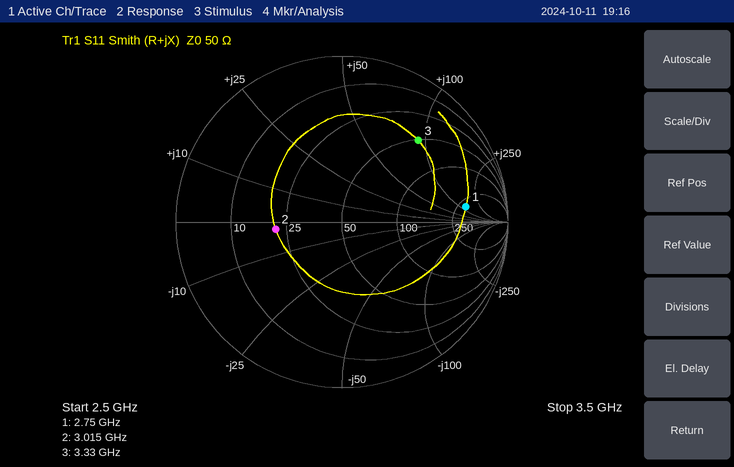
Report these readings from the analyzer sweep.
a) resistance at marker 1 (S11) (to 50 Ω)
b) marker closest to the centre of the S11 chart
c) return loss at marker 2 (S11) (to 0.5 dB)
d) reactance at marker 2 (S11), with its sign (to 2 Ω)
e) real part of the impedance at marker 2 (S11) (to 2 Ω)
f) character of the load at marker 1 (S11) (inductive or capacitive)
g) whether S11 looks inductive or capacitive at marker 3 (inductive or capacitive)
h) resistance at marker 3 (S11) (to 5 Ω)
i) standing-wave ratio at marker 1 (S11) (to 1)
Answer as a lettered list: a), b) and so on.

a) 300 Ω
b) marker 2
c) 8.0 dB
d) -2 Ω
e) 22 Ω
f) inductive
g) inductive
h) 50 Ω
i) 7
